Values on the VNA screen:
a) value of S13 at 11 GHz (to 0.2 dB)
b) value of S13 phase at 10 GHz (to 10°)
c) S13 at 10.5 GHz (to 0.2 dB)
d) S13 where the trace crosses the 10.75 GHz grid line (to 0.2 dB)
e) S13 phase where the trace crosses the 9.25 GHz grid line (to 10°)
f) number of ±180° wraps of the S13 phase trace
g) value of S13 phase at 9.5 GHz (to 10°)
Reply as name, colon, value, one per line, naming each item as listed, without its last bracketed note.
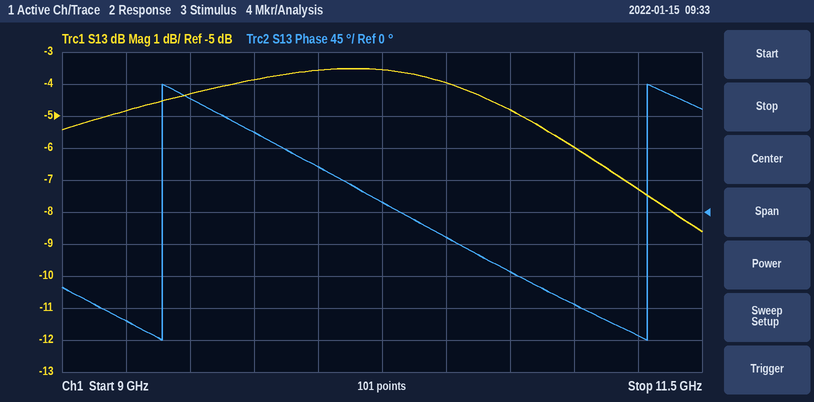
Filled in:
value of S13 at 11 GHz: -6.0 dB
value of S13 phase at 10 GHz: 60°
S13 at 10.5 GHz: -4.0 dB
S13 where the trace crosses the 10.75 GHz grid line: -4.8 dB
S13 phase where the trace crosses the 9.25 GHz grid line: -150°
number of ±180° wraps of the S13 phase trace: 2
value of S13 phase at 9.5 GHz: 160°
